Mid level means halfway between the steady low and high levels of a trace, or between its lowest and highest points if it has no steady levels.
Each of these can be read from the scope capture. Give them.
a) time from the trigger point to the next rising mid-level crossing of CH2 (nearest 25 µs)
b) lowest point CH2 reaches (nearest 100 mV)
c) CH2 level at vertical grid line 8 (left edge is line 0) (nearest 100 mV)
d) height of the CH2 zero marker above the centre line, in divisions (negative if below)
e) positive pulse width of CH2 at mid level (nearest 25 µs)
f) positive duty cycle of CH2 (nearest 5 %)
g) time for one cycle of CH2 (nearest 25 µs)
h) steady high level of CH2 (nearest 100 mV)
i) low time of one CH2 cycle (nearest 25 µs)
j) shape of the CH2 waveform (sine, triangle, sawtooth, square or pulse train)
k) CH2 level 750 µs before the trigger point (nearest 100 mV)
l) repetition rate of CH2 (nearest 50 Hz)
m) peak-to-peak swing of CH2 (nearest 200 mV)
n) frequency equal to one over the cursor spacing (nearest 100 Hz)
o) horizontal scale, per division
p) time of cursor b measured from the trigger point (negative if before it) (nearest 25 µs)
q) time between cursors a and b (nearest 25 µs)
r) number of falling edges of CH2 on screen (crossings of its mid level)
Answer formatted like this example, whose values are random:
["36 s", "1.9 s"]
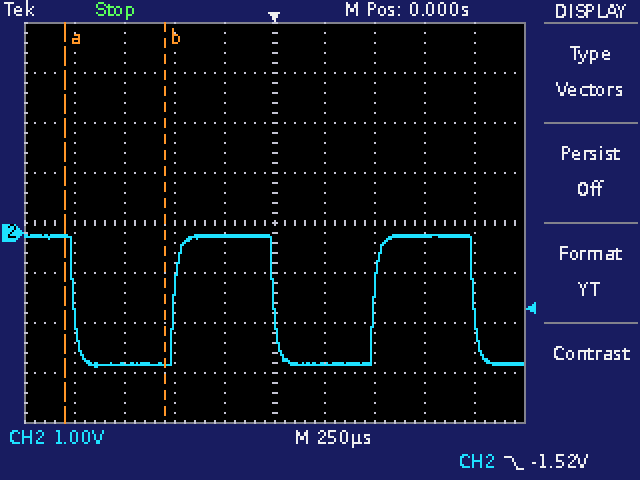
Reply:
["500 µs", "-2.7 V", "-100 mV", "-0.2 div", "500 µs", "50 %", "1.000 ms", "-100 mV", "500 µs", "square", "-2.6 V", "1.00 kHz", "2.6 V", "2.0 kHz", "250 µs", "-550 µs", "500 µs", "3"]
